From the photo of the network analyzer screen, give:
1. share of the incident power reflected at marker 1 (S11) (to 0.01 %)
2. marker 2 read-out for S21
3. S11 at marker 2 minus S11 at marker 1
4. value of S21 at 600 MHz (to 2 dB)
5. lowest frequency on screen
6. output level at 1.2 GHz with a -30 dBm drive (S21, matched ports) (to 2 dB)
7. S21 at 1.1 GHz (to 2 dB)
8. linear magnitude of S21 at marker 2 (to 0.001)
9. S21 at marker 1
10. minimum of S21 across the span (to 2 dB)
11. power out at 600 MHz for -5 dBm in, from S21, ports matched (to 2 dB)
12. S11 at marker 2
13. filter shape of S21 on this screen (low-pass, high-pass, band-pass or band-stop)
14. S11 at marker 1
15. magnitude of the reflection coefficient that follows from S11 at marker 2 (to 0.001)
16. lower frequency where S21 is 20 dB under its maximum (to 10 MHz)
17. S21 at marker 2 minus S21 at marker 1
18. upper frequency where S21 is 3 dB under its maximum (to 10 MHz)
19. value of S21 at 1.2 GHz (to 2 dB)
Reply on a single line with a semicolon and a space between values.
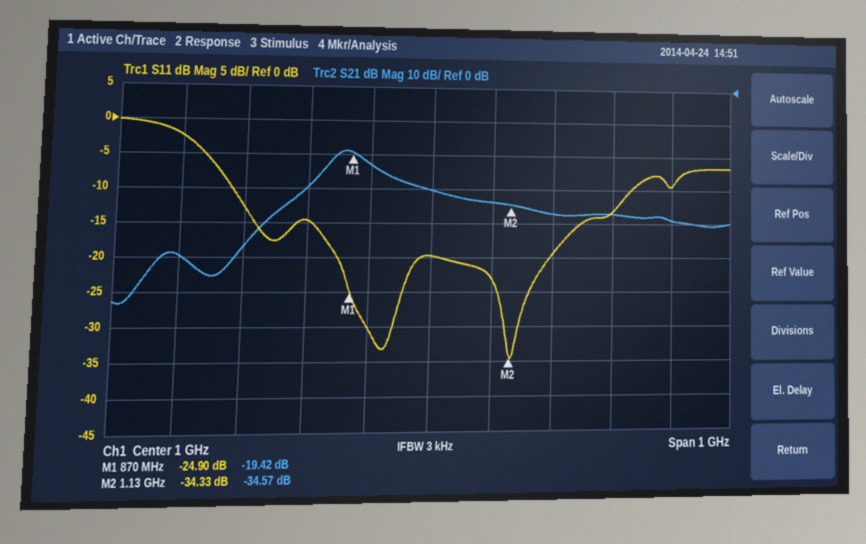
0.32 %; -34.57 dB; -9.43 dB; -50 dB; 500 MHz; -68 dBm; -34 dB; 0.019; -19.42 dB; -64 dB; -54 dBm; -34.33 dB; band-pass; -24.90 dB; 0.019; 740 MHz; -15.15 dB; 890 MHz; -38 dB
